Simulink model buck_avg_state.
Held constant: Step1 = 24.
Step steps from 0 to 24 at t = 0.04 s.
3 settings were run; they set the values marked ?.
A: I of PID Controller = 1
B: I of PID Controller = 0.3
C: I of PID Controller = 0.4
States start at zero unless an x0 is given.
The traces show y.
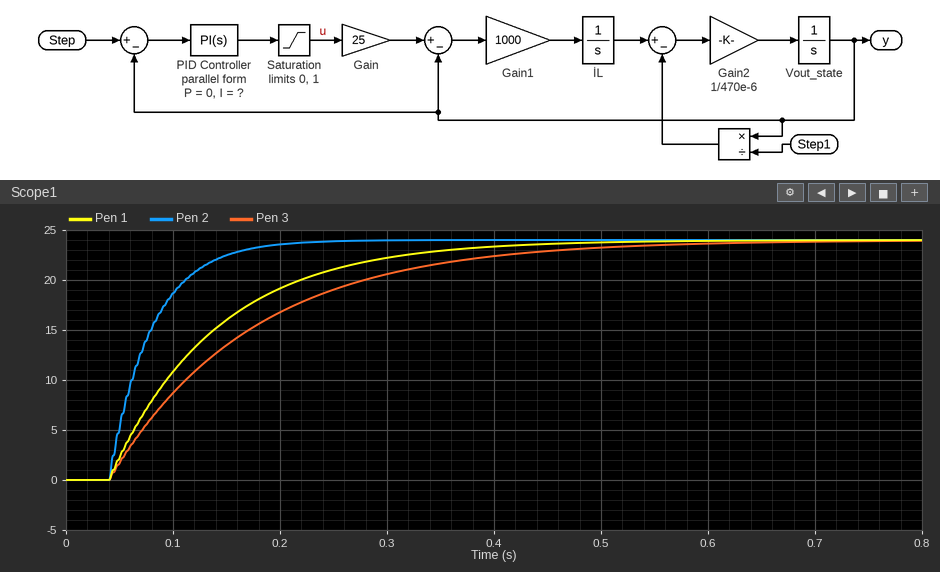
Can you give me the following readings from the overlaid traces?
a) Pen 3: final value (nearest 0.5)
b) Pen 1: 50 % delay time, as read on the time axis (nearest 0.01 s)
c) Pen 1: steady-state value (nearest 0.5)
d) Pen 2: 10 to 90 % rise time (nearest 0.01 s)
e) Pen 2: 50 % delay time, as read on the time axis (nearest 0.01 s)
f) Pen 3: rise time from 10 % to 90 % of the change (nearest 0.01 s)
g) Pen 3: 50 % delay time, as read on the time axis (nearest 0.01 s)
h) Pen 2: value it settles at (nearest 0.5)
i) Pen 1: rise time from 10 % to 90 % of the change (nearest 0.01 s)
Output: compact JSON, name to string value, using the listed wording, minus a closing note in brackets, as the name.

{"Pen 3: final value": "24.0", "Pen 1: 50 % delay time, as read on the time axis": "0.11 s", "Pen 1: steady-state value": "24.0", "Pen 2: 10 to 90 % rise time": "0.09 s", "Pen 2: 50 % delay time, as read on the time axis": "0.07 s", "Pen 3: rise time from 10 % to 90 % of the change": "0.29 s", "Pen 3: 50 % delay time, as read on the time axis": "0.13 s", "Pen 2: value it settles at": "24.0", "Pen 1: rise time from 10 % to 90 % of the change": "0.22 s"}
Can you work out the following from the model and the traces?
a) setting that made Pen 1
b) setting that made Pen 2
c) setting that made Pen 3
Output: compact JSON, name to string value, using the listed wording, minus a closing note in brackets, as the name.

{"setting that made Pen 1": "C", "setting that made Pen 2": "A", "setting that made Pen 3": "B"}
